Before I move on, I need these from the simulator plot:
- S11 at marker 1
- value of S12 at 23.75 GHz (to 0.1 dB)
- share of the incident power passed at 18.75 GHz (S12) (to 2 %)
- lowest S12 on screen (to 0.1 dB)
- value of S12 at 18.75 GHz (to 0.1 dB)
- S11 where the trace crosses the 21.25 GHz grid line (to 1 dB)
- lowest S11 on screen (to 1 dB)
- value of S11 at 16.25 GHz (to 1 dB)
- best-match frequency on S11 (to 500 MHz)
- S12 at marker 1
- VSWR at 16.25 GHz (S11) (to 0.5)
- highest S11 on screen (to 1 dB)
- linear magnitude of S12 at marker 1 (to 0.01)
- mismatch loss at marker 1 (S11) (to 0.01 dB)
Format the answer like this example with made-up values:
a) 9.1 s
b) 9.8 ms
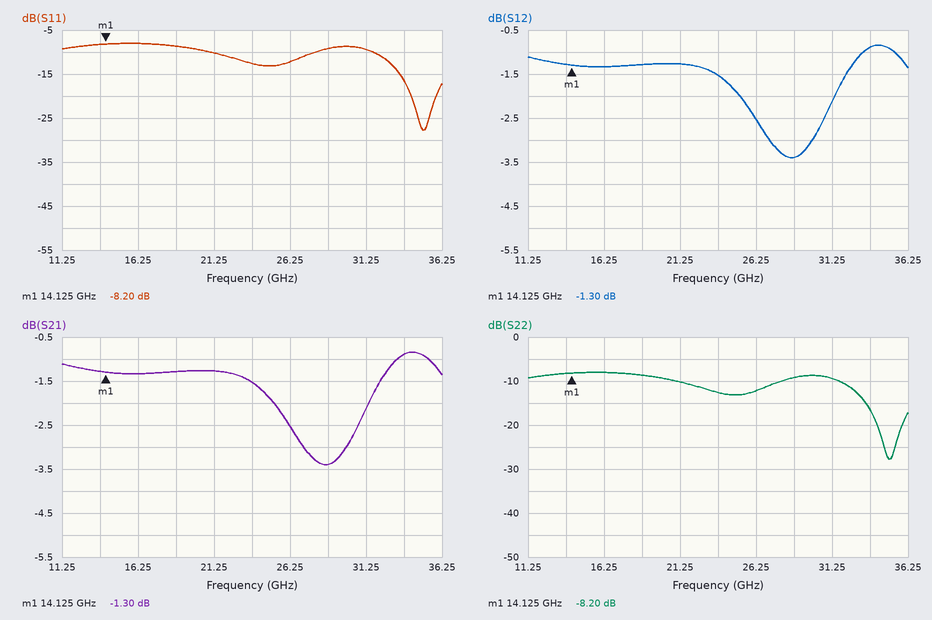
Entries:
a) -8.20 dB
b) -1.5 dB
c) 74 %
d) -3.4 dB
e) -1.3 dB
f) -10 dB
g) -28 dB
h) -8 dB
i) 35.0 GHz
j) -1.30 dB
k) 2.5
l) -8 dB
m) 0.86
n) 0.71 dB
